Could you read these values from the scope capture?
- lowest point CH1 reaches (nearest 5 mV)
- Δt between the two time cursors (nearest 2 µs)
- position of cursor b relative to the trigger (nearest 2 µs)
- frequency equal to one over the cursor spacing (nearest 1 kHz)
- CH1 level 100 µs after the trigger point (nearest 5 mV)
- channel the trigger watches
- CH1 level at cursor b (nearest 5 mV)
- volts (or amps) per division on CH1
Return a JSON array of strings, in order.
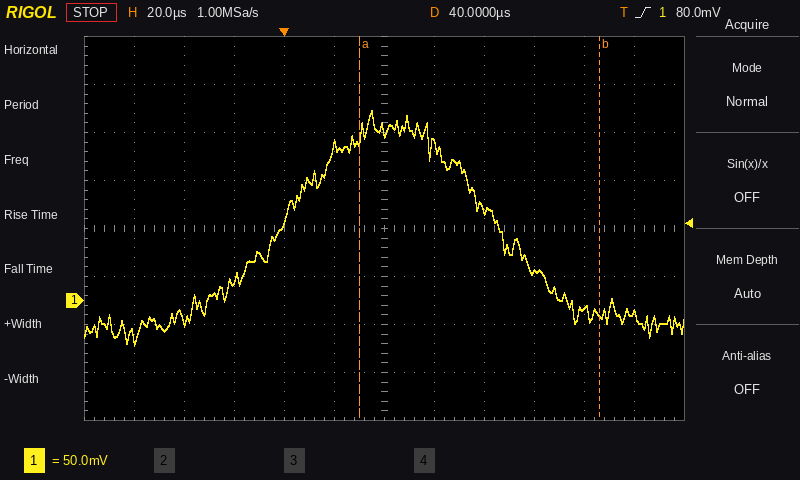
["-45 mV", "96 µs", "+126 µs", "10 kHz", "30 mV", "CH1", "-15 mV", "50 mV"]
